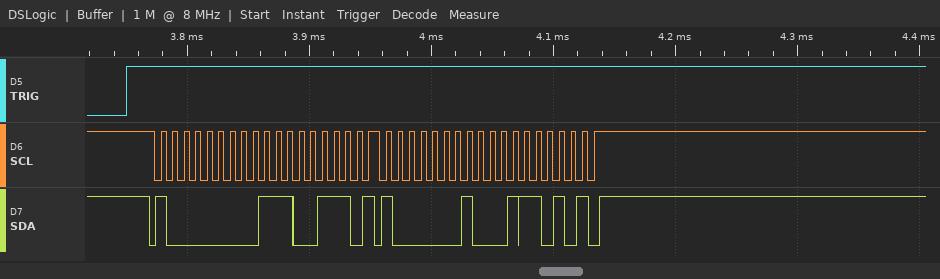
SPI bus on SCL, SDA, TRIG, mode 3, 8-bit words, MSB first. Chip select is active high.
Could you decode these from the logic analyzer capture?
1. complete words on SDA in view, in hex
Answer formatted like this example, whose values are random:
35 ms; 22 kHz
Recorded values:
80, 73, B0, 23
